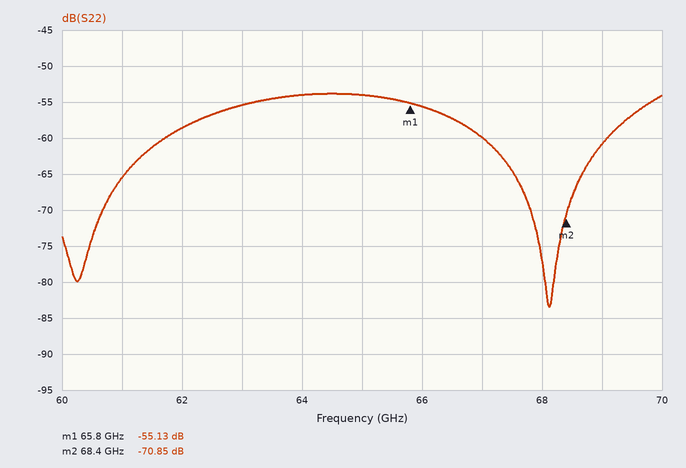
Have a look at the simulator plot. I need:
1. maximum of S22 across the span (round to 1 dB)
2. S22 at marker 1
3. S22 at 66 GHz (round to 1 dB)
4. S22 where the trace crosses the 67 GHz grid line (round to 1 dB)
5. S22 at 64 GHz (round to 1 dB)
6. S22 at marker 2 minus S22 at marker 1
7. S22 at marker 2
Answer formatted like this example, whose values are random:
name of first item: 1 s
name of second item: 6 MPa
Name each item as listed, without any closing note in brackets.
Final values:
maximum of S22 across the span: -54 dB
S22 at marker 1: -55.13 dB
S22 at 66 GHz: -56 dB
S22 where the trace crosses the 67 GHz grid line: -60 dB
S22 at 64 GHz: -54 dB
S22 at marker 2 minus S22 at marker 1: -15.72 dB
S22 at marker 2: -70.85 dB
